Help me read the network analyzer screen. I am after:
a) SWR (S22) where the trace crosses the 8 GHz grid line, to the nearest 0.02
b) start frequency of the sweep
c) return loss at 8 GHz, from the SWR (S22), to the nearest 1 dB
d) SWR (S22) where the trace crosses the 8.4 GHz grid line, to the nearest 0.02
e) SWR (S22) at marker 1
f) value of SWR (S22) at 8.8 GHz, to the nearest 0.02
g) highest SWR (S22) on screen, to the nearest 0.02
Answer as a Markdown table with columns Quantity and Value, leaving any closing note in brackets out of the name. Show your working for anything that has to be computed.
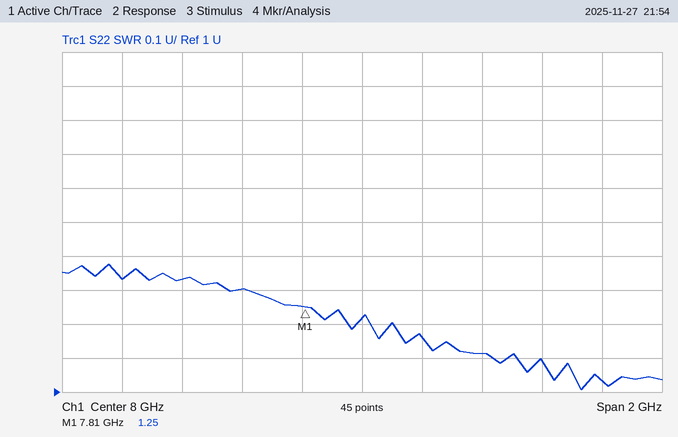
| Quantity | Value |
|---|---|
| SWR (S22) where the trace crosses the 8 GHz grid line, to the nearest 0.02 | 1.22 |
| start frequency of the sweep | 7 GHz |
| return loss at 8 GHz, from the SWR (S22), to the nearest 1 dB | −20 log10((1.22 − 1)/(1.22 + 1)) ≈ 20 dB |
| SWR (S22) where the trace crosses the 8.4 GHz grid line, to the nearest 0.02 | 1.12 |
| SWR (S22) at marker 1 | 1.25 |
| value of SWR (S22) at 8.8 GHz, to the nearest 0.02 | 1.04 |
| highest SWR (S22) on screen, to the nearest 0.02 | 1.38 |
